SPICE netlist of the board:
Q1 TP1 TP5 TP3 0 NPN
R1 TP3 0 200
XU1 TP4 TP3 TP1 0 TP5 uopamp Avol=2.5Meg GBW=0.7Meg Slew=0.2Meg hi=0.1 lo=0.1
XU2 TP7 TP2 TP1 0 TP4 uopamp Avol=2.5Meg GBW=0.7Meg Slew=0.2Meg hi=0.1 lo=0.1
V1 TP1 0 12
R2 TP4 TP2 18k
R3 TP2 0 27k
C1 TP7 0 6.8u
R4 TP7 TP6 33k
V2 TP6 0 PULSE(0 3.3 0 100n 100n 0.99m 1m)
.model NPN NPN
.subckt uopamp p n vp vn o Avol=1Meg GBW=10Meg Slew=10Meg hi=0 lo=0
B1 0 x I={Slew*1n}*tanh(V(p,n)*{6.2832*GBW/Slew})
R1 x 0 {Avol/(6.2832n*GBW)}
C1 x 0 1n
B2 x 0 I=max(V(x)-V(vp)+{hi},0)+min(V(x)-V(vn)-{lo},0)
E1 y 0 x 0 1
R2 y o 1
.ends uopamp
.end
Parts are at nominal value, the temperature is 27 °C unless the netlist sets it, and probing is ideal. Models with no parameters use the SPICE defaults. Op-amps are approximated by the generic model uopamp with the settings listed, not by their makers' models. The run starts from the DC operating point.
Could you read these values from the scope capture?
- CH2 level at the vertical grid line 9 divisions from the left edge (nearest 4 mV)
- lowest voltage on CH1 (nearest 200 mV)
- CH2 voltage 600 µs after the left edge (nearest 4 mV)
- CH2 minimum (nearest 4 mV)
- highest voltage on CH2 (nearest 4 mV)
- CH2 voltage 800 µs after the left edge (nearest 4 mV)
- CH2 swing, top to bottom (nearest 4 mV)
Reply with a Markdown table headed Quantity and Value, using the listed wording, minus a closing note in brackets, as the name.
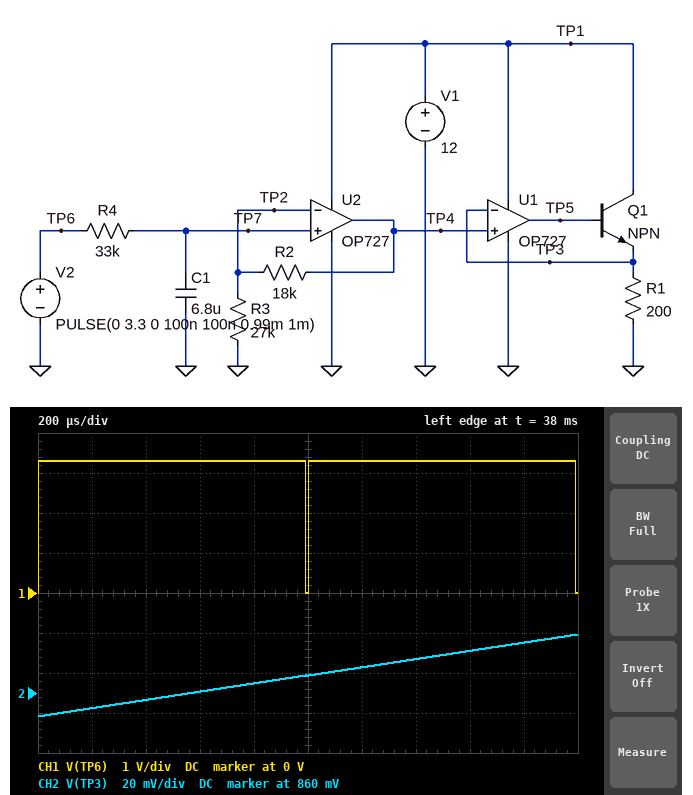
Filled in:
| Quantity | Value |
|---|---|
| CH2 level at the vertical grid line 9 divisions from the left edge | 884 mV |
| lowest voltage on CH1 | 0 V |
| CH2 voltage 600 µs after the left edge | 860 mV |
| CH2 minimum | 848 mV |
| highest voltage on CH2 | 888 mV |
| CH2 voltage 800 µs after the left edge | 864 mV |
| CH2 swing, top to bottom | 40 mV |
